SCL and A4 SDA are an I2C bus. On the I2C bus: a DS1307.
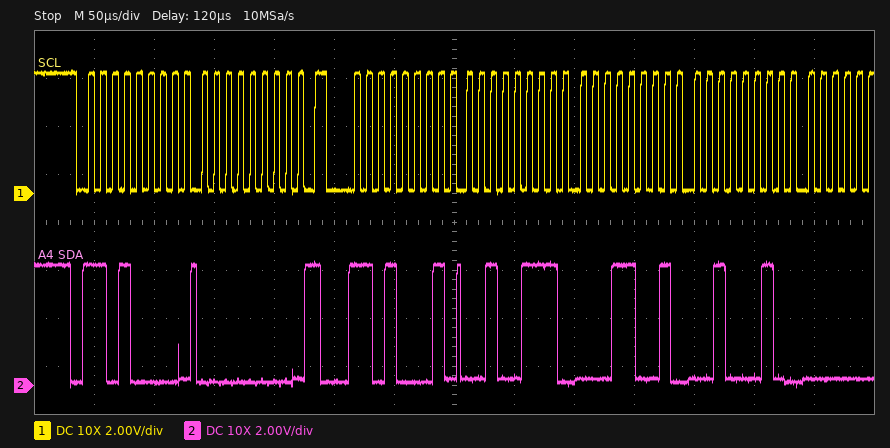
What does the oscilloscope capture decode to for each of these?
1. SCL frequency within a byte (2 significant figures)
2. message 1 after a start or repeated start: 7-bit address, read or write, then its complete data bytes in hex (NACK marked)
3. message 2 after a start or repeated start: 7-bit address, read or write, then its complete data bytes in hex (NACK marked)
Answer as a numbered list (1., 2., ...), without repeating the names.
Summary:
1. 100 kHz
2. 0x68 write: 00
3. 0x68 read: 27 19 22
